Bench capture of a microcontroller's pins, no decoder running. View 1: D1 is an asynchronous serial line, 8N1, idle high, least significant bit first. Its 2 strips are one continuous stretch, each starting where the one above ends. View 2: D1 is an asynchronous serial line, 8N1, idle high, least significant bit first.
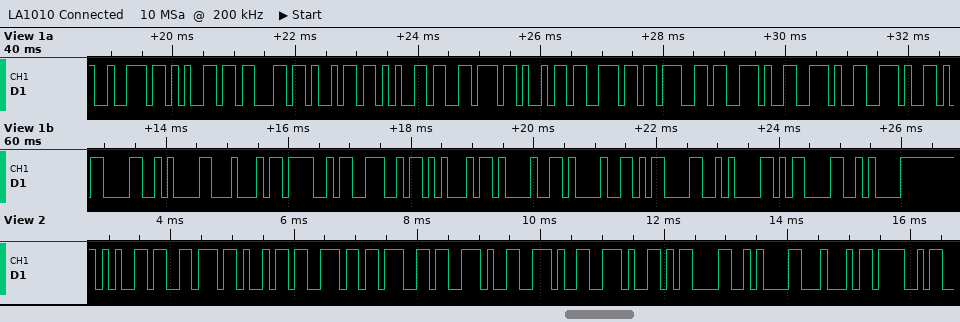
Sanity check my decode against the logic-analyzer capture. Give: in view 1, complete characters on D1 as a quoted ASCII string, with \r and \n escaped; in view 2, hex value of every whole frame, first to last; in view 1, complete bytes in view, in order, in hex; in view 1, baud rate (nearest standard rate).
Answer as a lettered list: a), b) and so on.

a) "recieving...\r\nDONE!!\r\n\r\n"
b) 65 76 69 6E 67 2E 2E 2E 0D 0A 44 4F
c) 0x72 0x65 0x63 0x69 0x65 0x76 0x69 0x6E 0x67 0x2E 0x2E 0x2E 0x0D 0x0A 0x44 0x4F 0x4E 0x45 0x21 0x21 0x0D 0x0A 0x0D 0x0A
d) 9600 baud
